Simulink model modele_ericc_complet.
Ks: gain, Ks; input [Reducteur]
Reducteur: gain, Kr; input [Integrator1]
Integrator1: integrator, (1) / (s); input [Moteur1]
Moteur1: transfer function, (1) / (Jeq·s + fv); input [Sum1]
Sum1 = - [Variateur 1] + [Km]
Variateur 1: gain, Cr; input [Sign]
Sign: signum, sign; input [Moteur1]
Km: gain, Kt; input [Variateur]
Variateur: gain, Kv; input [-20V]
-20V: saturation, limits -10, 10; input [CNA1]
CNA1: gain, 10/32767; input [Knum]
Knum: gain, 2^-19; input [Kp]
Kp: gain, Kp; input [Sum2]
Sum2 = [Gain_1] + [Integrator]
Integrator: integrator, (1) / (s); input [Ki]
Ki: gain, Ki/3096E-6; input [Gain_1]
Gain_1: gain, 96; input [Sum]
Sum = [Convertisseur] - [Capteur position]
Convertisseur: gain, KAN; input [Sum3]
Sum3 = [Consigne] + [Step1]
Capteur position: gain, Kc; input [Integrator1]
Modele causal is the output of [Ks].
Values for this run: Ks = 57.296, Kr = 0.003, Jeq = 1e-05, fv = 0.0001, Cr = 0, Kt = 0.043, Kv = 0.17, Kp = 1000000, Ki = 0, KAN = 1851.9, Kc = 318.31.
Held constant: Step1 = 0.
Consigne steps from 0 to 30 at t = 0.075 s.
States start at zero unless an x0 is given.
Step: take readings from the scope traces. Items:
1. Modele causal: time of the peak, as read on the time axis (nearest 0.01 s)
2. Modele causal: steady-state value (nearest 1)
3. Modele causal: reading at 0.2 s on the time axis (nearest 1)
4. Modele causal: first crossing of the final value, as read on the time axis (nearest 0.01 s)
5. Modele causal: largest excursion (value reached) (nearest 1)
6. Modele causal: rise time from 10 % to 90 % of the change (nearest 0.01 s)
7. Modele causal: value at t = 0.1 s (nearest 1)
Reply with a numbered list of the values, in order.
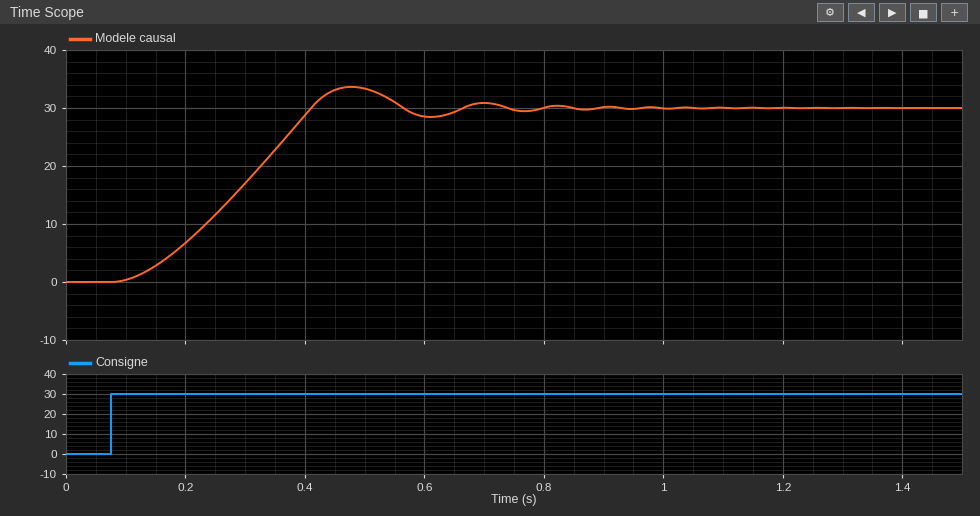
1. 0.48 s
2. 30
3. 7
4. 0.41 s
5. 34
6. 0.23 s
7. 0
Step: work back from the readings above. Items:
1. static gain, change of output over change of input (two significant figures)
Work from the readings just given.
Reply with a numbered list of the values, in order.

1. 1.0
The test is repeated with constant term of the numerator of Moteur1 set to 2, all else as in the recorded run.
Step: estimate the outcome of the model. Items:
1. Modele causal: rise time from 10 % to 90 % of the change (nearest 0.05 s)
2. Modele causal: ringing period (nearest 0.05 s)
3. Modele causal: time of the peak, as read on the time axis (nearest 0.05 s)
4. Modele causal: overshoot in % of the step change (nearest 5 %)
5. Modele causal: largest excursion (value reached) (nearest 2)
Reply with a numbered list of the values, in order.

1. 0.15 s
2. 0.20 s
3. 0.35 s
4. 20 %
5. 36
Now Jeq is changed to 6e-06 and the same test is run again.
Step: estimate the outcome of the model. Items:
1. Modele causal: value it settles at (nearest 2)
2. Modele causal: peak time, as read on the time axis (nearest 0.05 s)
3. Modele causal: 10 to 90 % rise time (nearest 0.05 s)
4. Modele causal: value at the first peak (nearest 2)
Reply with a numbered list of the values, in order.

1. 30
2. 0.40 s
3. 0.20 s
4. 32
